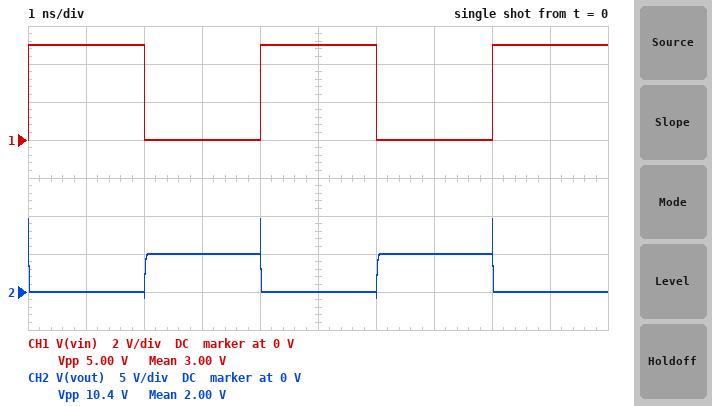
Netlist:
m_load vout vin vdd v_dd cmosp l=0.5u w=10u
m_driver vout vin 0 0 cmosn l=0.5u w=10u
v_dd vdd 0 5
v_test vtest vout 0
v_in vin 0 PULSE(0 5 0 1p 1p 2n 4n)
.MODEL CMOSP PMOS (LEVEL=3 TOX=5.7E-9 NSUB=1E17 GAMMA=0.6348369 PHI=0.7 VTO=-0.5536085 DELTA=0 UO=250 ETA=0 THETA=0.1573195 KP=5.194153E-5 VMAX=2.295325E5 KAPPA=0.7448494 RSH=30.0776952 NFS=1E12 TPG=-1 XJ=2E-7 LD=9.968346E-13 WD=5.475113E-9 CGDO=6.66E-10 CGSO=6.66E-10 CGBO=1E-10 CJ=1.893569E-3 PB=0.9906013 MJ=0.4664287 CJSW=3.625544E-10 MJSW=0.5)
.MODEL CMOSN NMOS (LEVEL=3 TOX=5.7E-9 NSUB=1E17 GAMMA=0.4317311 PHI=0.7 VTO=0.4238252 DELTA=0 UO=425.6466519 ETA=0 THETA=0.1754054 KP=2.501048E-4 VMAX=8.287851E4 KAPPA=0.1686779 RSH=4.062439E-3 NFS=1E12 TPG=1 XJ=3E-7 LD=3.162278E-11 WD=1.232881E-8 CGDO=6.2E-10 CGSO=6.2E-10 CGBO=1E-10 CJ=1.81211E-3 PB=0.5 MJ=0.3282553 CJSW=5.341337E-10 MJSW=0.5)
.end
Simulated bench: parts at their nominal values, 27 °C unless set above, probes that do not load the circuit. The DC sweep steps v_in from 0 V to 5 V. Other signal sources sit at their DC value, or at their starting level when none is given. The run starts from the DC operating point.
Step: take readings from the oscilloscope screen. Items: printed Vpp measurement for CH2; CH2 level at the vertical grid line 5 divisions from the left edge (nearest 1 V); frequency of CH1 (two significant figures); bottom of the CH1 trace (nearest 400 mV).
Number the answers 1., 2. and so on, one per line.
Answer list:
1. 10.4 V
2. 0 V
3. 250 MHz
4. 0 V
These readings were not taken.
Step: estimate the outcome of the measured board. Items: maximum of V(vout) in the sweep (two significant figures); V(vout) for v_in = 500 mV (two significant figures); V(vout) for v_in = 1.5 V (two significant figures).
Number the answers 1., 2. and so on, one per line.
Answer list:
1. 5.0 V
2. 5.0 V
3. 3.8 V
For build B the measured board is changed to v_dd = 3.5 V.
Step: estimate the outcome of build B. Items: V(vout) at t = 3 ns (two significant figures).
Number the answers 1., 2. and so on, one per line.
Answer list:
1. 3.5 V
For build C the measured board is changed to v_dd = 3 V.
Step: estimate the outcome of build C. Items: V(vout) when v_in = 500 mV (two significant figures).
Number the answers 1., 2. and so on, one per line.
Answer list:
1. 3.0 V
